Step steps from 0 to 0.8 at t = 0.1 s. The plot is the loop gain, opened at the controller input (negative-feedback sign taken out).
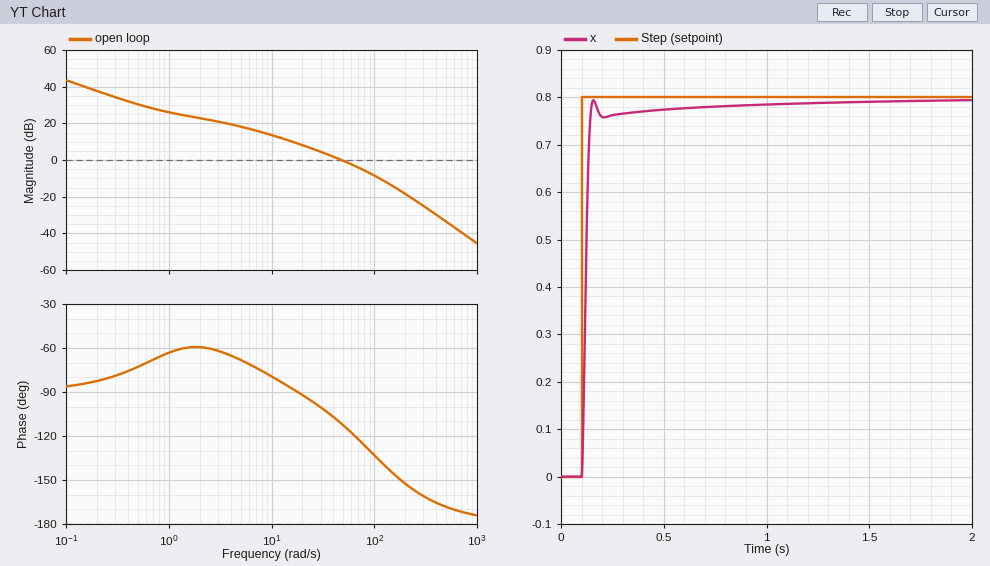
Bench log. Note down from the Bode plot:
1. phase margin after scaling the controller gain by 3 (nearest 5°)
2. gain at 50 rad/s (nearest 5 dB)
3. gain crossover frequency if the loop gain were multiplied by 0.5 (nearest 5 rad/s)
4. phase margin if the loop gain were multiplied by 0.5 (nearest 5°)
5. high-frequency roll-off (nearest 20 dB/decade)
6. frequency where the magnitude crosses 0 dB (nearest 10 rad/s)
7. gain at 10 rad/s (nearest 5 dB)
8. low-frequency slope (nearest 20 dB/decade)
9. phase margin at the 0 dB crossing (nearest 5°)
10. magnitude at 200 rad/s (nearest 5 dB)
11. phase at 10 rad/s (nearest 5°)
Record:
45°
0 dB
25 rad/s
85°
-40 dB/decade
50 rad/s
15 dB
-20 dB/decade
70°
-20 dB
-80°
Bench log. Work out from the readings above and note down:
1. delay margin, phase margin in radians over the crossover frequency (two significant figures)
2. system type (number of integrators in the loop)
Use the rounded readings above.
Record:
0.024 s
1
